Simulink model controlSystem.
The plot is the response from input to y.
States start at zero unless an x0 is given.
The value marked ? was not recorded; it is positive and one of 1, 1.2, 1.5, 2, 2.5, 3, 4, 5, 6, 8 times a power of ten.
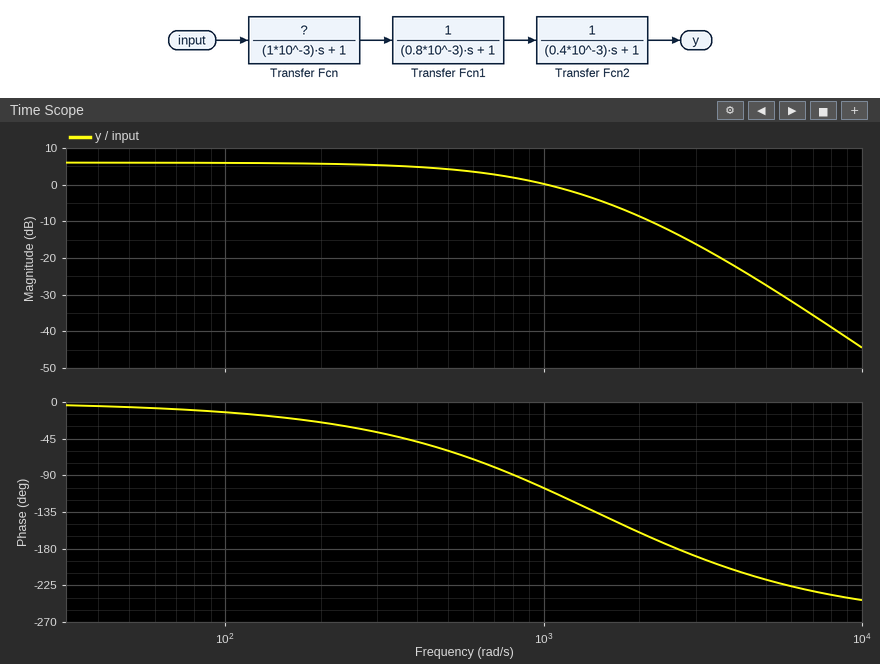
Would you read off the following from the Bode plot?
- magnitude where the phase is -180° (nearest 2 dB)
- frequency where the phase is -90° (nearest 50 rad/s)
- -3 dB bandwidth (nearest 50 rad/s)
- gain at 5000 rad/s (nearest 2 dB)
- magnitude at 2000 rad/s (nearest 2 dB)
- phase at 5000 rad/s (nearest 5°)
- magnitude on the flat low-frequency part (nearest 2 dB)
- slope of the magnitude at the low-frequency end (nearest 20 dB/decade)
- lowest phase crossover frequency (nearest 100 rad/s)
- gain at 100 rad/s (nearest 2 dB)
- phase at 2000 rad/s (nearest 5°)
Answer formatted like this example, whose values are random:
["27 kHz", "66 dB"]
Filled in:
["-14 dB", "800 rad/s", "650 rad/s", "-28 dB", "-8 dB", "-220°", "6 dB", "0 dB/decade", "2600 rad/s", "6 dB", "-160°"]
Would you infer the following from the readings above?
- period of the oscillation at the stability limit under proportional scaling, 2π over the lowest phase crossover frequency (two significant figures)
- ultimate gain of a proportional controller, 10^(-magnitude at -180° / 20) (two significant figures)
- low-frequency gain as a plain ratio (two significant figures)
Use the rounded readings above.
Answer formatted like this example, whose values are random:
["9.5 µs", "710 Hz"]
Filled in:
["0.0024 s", "5.0", "2.0"]
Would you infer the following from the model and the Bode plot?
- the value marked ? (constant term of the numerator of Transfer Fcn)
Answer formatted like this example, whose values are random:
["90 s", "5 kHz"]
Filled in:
["2"]
